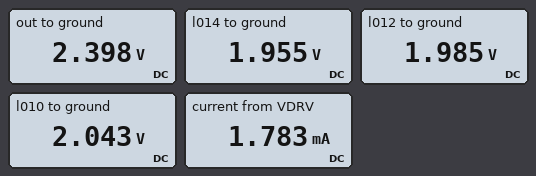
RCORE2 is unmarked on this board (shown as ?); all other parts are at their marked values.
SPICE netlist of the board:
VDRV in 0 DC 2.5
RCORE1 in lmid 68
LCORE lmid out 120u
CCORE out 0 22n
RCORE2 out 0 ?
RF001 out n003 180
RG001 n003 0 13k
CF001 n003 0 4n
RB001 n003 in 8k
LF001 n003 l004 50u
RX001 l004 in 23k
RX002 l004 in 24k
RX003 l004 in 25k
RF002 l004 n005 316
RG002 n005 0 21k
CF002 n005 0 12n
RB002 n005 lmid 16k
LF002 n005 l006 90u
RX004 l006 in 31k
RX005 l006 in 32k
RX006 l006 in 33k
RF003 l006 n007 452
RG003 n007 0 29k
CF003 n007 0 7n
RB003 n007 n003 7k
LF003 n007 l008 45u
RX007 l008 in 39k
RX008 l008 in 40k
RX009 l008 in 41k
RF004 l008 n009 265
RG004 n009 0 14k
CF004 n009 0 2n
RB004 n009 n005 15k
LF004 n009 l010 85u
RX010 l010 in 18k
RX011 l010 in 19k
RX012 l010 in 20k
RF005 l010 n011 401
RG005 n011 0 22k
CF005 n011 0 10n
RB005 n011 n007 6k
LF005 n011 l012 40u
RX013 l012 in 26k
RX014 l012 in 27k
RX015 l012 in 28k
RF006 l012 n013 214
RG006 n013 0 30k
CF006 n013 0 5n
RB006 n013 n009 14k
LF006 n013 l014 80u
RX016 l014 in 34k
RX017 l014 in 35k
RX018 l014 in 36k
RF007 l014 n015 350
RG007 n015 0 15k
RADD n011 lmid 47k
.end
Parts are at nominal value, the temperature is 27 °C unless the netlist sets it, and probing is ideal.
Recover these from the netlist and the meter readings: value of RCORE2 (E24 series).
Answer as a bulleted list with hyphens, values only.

- 2.4 kΩ
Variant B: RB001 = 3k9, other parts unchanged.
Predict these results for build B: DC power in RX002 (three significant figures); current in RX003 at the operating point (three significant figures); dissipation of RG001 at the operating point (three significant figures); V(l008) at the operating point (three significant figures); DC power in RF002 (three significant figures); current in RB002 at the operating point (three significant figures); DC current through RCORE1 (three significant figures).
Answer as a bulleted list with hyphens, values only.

- 1.41 µW
- 7.36 µA
- 413 µW
- 2.10 V
- 33.2 µW
- 11.6 µA
- 1.48 mA
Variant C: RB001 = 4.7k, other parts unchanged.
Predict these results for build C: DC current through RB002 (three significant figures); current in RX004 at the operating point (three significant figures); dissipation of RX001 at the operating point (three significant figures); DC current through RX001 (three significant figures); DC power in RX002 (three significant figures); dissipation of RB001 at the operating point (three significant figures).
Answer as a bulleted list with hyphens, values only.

- 11.7 µA
- 9.28 µA
- 1.50 µW
- 8.07 µA
- 1.44 µW
- 7.33 µW
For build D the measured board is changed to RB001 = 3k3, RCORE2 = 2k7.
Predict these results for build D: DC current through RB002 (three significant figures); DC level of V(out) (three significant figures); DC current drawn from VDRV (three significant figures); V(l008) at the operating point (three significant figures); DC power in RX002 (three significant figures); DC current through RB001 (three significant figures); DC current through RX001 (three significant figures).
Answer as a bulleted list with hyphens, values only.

- 11.7 µA
- 2.41 V
- 1.68 mA
- 2.11 V
- 1.30 µW
- 53.5 µA
- 7.67 µA
